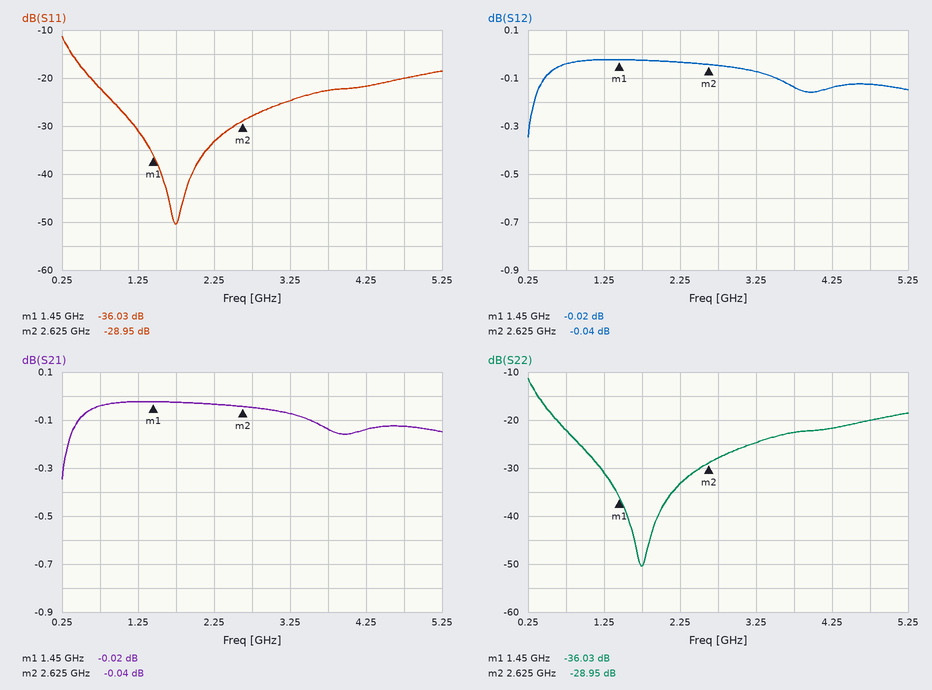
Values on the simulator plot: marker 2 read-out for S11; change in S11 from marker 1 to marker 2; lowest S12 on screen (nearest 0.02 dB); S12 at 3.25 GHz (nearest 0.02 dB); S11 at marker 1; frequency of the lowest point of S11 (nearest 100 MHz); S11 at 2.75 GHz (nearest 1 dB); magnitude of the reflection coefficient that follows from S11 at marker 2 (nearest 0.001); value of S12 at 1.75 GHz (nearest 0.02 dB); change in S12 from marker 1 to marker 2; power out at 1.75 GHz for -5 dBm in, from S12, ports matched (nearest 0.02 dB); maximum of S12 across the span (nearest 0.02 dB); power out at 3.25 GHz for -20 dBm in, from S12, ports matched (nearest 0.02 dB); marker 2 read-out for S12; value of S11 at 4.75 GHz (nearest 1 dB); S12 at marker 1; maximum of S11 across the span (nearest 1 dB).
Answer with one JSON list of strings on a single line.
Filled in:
["-28.95 dB", "7.08 dB", "-0.34 dB", "-0.08 dB", "-36.03 dB", "1.7 GHz", "-28 dB", "0.036", "-0.02 dB", "-0.02 dB", "-5.02 dBm", "-0.02 dB", "-20.08 dBm", "-0.04 dB", "-20 dB", "-0.02 dB", "-11 dB"]
